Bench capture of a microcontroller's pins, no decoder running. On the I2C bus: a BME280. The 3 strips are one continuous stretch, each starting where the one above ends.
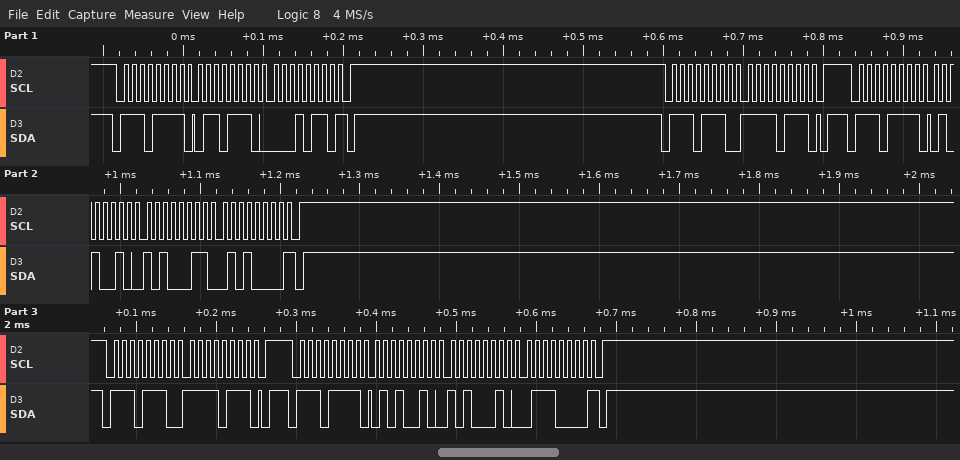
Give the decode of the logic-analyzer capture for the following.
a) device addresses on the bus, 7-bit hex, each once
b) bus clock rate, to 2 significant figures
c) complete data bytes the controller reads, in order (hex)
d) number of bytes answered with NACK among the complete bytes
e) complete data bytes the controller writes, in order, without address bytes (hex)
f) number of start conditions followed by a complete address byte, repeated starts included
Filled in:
0x77
100 kHz
6E 16 52 A3 50 52 A2 70
3
F7 F7
5
